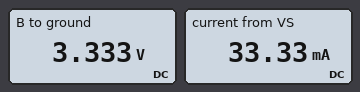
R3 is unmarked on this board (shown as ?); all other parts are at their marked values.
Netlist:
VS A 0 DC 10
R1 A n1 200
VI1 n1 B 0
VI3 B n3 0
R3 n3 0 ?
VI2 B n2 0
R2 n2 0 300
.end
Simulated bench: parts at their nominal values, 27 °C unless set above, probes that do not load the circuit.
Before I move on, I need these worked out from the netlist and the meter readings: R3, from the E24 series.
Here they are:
150 Ω
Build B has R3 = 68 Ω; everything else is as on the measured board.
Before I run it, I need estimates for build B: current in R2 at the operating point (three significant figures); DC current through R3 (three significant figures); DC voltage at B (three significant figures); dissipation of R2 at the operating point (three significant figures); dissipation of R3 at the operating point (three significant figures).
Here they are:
7.23 mA
31.9 mA
2.17 V
15.7 mW
69.3 mW
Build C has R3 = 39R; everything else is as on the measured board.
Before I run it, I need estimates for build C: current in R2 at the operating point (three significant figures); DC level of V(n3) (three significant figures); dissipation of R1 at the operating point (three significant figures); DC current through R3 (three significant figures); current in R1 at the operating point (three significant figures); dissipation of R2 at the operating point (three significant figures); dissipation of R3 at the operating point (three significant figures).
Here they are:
4.91 mA
1.47 V
364 mW
37.7 mA
42.6 mA
7.22 mW
55.5 mW
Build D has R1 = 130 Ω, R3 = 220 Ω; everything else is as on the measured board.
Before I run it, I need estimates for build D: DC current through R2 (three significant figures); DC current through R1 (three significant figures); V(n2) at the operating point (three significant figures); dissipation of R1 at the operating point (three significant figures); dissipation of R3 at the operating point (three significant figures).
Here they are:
16.5 mA
38.9 mA
4.94 V
197 mW
111 mW
